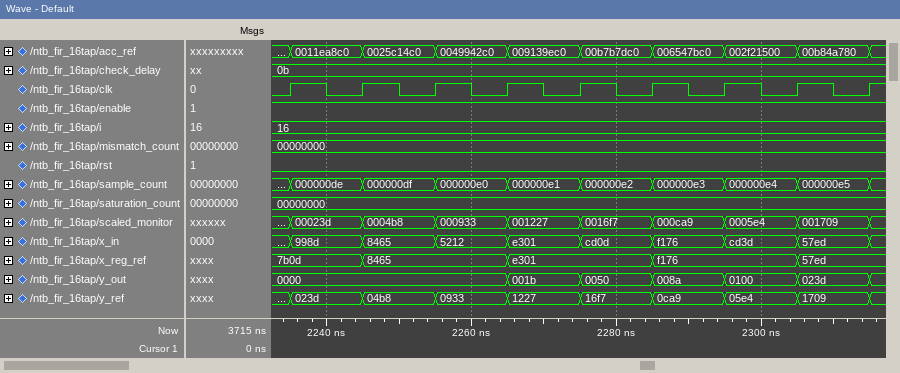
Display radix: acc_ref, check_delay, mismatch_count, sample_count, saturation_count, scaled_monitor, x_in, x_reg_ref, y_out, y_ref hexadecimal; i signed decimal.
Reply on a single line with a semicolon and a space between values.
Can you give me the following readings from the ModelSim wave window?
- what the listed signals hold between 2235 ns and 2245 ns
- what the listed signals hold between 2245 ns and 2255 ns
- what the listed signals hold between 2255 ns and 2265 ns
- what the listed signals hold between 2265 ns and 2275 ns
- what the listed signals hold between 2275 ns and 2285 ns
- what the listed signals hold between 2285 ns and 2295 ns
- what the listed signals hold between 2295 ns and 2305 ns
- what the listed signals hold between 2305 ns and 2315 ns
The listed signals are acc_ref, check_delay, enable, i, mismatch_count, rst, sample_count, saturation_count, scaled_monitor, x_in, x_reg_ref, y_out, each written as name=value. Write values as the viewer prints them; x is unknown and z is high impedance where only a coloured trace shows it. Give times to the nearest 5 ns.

acc_ref=0011ea8c0, check_delay=0b, enable=1, i=16, mismatch_count=00000000, rst=0, sample_count=000000de, saturation_count=00000000, scaled_monitor=00023d, x_in=998d, x_reg_ref=7b0d, y_out=0000; acc_ref=0025c14c0, check_delay=0b, enable=1, i=16, mismatch_count=00000000, rst=0, sample_count=000000df, saturation_count=00000000, scaled_monitor=0004b8, x_in=8465, x_reg_ref=8465, y_out=0000; acc_ref=0049942c0, check_delay=0b, enable=1, i=16, mismatch_count=00000000, rst=0, sample_count=000000e0, saturation_count=00000000, scaled_monitor=000933, x_in=5212, x_reg_ref=8465, y_out=0000; acc_ref=009139ec0, check_delay=0b, enable=1, i=16, mismatch_count=00000000, rst=0, sample_count=000000e1, saturation_count=00000000, scaled_monitor=001227, x_in=e301, x_reg_ref=e301, y_out=001b; acc_ref=00b7b7dc0, check_delay=0b, enable=1, i=16, mismatch_count=00000000, rst=0, sample_count=000000e2, saturation_count=00000000, scaled_monitor=0016f7, x_in=cd0d, x_reg_ref=e301, y_out=0050; acc_ref=006547bc0, check_delay=0b, enable=1, i=16, mismatch_count=00000000, rst=0, sample_count=000000e3, saturation_count=00000000, scaled_monitor=000ca9, x_in=f176, x_reg_ref=f176, y_out=008a; acc_ref=002f21500, check_delay=0b, enable=1, i=16, mismatch_count=00000000, rst=0, sample_count=000000e4, saturation_count=00000000, scaled_monitor=0005e4, x_in=cd3d, x_reg_ref=f176, y_out=0100; acc_ref=00b84a780, check_delay=0b, enable=1, i=16, mismatch_count=00000000, rst=0, sample_count=000000e5, saturation_count=00000000, scaled_monitor=001709, x_in=57ed, x_reg_ref=57ed, y_out=023d
